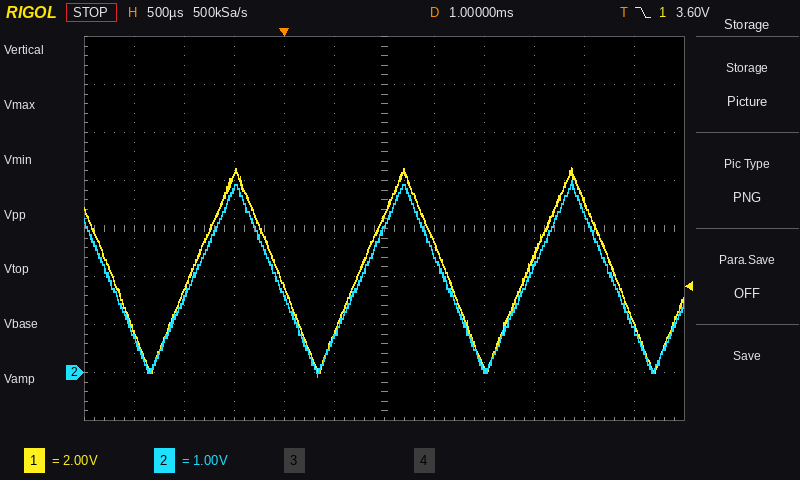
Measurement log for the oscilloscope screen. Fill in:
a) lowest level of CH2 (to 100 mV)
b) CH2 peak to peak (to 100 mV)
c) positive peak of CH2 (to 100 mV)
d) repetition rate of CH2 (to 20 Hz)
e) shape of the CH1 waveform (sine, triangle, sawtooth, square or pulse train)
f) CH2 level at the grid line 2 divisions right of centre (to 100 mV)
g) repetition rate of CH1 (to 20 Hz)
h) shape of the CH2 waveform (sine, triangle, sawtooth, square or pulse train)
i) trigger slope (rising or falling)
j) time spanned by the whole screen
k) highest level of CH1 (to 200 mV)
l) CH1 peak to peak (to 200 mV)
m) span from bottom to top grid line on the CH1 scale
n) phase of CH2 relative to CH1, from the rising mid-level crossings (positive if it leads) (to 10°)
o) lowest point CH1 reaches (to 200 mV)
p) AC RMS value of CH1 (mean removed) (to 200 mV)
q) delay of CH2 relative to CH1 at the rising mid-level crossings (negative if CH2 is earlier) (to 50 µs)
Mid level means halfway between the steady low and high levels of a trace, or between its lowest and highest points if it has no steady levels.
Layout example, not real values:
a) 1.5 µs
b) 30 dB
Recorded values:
a) -100 mV
b) 4.1 V
c) 4.0 V
d) 600 Hz
e) triangle
f) 100 mV
g) 600 Hz
h) triangle
i) falling
j) 6 ms
k) 8.6 V
l) 8.6 V
m) 16 V
n) 0°
o) 0.0 V
p) 2.4 V
q) 0 µs
